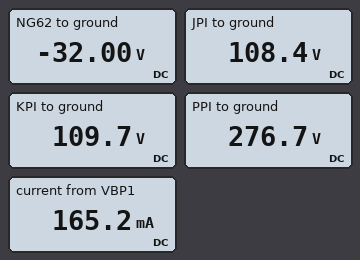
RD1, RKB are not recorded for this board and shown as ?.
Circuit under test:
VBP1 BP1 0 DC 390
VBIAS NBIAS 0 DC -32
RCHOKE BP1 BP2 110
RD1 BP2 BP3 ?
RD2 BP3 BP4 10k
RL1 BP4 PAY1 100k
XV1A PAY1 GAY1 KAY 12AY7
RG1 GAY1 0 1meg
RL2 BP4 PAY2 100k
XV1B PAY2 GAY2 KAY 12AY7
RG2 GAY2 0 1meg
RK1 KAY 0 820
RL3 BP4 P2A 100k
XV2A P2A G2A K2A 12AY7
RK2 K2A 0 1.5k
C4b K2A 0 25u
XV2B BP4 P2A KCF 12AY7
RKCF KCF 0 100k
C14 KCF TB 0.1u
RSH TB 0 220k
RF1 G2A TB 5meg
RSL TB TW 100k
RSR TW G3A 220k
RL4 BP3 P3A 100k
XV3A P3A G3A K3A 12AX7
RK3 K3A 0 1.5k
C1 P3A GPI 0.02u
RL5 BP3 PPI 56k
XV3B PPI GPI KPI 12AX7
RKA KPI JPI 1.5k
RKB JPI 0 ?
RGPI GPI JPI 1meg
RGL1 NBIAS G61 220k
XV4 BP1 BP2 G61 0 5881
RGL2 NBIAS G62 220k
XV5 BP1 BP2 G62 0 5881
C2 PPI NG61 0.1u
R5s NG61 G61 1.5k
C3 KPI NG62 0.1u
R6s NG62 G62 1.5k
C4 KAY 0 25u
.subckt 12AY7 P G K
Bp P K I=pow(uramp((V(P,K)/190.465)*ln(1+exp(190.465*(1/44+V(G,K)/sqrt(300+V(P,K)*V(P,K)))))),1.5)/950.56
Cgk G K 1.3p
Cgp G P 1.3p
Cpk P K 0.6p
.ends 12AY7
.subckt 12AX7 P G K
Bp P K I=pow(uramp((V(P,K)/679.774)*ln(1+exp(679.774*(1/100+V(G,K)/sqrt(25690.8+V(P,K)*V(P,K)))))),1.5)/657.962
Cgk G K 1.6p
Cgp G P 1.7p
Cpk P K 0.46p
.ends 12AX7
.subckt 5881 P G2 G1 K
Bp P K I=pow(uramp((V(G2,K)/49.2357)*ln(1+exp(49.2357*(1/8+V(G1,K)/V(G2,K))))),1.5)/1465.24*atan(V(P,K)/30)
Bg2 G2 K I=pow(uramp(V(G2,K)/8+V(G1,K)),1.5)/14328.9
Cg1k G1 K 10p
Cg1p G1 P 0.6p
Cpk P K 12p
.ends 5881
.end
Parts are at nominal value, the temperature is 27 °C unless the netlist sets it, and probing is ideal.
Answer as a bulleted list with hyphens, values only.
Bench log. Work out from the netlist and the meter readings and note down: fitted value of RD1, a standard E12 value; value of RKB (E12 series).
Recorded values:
- 8.2 kΩ
- 120 kΩ
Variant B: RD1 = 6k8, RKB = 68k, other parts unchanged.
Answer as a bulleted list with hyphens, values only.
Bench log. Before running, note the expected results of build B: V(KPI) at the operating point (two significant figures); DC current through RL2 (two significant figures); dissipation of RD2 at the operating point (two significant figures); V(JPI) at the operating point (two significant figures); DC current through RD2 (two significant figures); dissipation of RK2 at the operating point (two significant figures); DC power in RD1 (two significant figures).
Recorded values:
- 74 V
- 1.4 mA
- 310 mW
- 72 V
- 5.5 mA
- 2.9 mW
- 410 mW
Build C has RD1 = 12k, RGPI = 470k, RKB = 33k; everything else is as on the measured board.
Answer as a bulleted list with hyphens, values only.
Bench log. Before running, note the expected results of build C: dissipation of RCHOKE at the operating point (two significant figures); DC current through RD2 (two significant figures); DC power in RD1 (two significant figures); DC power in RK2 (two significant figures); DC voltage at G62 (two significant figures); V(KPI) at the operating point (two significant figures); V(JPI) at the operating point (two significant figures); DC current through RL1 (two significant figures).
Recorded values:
- 30 mW
- 5.0 mA
- 610 mW
- 2.4 mW
- -32 V
- 37 V
- 36 V
- 1.2 mA
